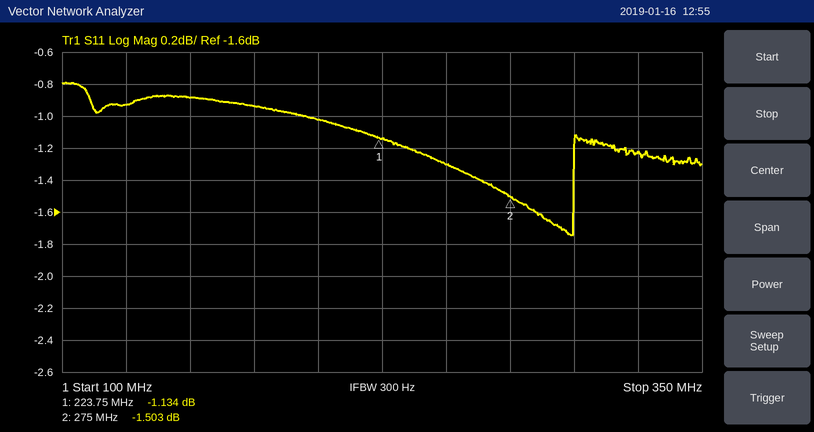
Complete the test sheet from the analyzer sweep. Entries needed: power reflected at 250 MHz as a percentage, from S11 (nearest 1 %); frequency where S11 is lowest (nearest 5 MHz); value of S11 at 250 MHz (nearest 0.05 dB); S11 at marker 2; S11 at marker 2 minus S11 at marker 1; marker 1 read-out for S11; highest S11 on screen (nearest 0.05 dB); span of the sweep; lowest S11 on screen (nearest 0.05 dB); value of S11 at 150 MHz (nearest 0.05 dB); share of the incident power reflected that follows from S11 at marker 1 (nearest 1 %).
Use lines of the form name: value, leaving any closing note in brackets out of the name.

power reflected at 250 MHz as a percentage, from S11: 74 %
frequency where S11 is lowest: 300 MHz
value of S11 at 250 MHz: -1.30 dB
S11 at marker 2: -1.503 dB
S11 at marker 2 minus S11 at marker 1: -0.369 dB
marker 1 read-out for S11: -1.134 dB
highest S11 on screen: -0.80 dB
span of the sweep: 250 MHz
lowest S11 on screen: -1.75 dB
value of S11 at 150 MHz: -0.90 dB
share of the incident power reflected that follows from S11 at marker 1: 77 %
